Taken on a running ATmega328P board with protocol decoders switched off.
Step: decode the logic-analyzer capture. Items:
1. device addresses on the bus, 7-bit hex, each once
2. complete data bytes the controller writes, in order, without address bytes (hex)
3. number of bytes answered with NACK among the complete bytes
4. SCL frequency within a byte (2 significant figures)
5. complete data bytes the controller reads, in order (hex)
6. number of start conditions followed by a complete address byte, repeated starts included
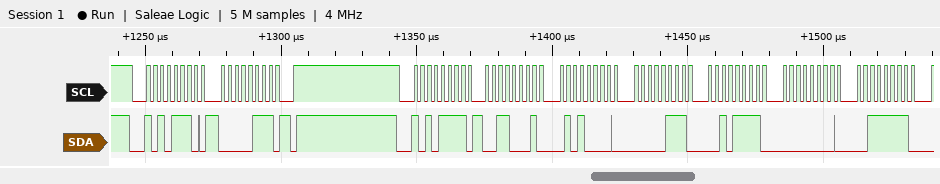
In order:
0x57
07
0
400 kHz
31 50 07 2F 00 3F
2
